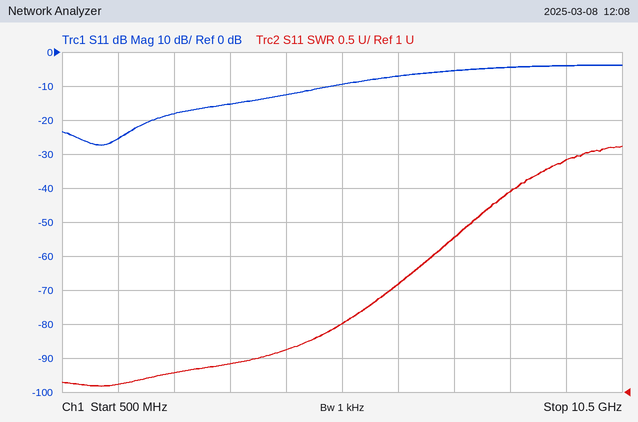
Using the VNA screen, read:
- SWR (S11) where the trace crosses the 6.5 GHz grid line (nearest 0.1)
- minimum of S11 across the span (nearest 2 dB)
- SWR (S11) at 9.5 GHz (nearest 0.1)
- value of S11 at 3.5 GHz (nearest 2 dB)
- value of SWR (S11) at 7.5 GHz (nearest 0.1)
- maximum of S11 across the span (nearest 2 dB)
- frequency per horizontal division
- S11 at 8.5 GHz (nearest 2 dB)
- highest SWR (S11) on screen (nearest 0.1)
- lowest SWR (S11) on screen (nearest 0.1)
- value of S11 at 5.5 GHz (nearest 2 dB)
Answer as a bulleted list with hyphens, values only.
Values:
- 2.6
- -28 dB
- 4.4
- -16 dB
- 3.3
- -4 dB
- 1 GHz
- -4 dB
- 4.6
- 1.1
- -10 dB
